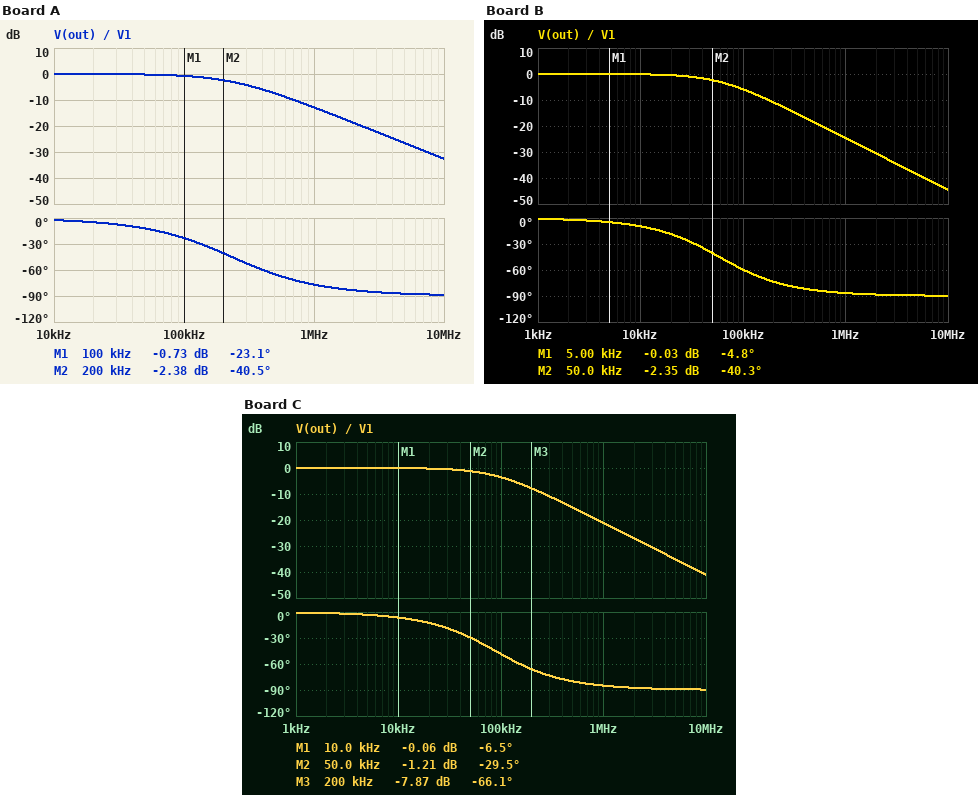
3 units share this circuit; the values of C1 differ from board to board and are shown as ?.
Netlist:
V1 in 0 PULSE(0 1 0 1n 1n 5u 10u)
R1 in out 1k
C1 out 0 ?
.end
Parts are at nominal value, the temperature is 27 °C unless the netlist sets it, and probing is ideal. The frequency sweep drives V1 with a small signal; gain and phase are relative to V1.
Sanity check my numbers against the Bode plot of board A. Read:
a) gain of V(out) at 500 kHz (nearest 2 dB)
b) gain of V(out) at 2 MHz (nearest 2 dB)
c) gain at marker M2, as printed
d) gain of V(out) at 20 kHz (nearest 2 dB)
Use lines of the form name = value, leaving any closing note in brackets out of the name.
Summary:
gain of V(out) at 500 kHz = -8 dB
gain of V(out) at 2 MHz = -18 dB
gain at marker M2, as printed = -2.38 dB
gain of V(out) at 20 kHz = 0 dB
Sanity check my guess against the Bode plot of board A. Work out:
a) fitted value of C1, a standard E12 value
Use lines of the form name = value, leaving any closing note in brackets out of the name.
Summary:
fitted value of C1, a standard E12 value = 680 pF
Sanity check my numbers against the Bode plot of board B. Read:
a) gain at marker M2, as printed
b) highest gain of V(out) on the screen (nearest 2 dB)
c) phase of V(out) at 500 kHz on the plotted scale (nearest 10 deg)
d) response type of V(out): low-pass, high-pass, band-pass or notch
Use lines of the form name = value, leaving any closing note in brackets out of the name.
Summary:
gain at marker M2, as printed = -2.35 dB
highest gain of V(out) on the screen = 0 dB
phase of V(out) at 500 kHz on the plotted scale = -80 deg
response type of V(out): low-pass, high-pass, band-pass or notch = low-pass
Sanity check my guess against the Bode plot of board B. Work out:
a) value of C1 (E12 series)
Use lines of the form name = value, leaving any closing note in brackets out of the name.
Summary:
value of C1 = 2.7 nF
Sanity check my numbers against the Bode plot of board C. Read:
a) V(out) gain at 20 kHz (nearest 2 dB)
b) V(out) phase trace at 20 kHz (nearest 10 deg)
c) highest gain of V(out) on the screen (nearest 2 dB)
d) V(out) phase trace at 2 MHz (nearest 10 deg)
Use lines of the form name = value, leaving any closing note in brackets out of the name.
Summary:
V(out) gain at 20 kHz = 0 dB
V(out) phase trace at 20 kHz = -10 deg
highest gain of V(out) on the screen = 0 dB
V(out) phase trace at 2 MHz = -90 deg
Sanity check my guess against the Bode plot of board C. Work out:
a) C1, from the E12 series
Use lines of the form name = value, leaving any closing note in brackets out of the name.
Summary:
C1, from the E12 series = 1.8 nF
